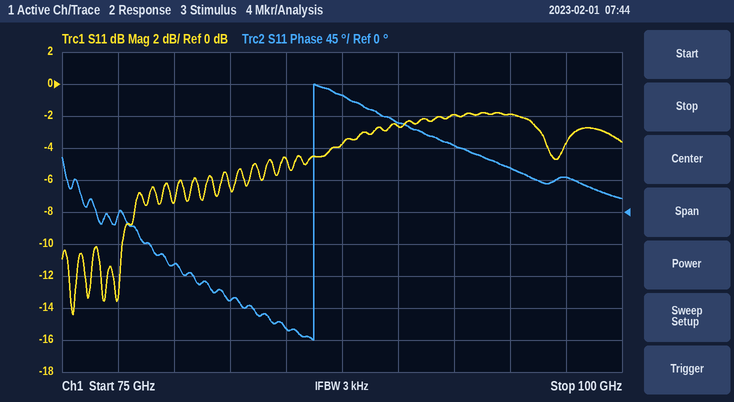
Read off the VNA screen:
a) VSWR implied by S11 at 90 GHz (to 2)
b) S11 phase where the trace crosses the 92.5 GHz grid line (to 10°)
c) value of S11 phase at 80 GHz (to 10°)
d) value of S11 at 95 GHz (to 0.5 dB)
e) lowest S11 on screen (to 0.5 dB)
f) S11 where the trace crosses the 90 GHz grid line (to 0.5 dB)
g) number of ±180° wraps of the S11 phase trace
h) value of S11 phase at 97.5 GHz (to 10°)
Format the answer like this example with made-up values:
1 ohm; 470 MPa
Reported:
6; 90°; -70°; -2.0 dB; -14.5 dB; -2.5 dB; 1; 50°
